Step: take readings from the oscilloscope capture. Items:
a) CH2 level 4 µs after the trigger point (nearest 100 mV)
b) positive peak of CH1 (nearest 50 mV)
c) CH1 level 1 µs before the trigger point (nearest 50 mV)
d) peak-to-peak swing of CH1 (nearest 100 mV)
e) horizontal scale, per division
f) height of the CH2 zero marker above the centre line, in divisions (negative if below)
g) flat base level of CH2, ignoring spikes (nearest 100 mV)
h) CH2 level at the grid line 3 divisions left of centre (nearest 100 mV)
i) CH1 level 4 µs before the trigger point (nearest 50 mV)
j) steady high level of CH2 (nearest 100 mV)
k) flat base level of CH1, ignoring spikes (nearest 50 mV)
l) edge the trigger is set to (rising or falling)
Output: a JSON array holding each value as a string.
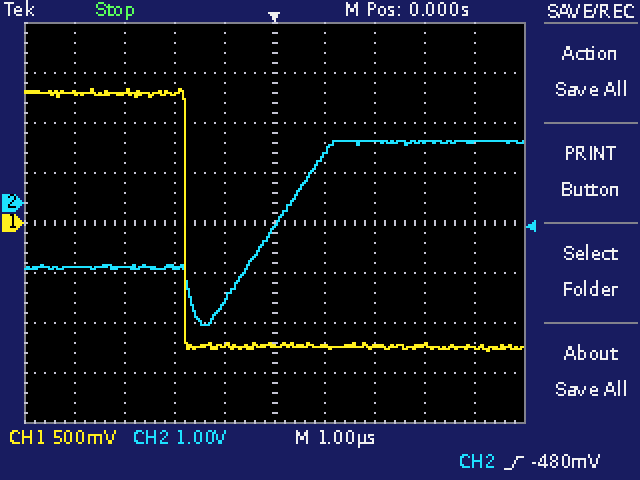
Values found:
["1.2 V", "1.35 V", "-1.20 V", "2.60 V", "1 µs", "+0.4 div", "-1.3 V", "-1.3 V", "1.30 V", "1.2 V", "-1.25 V", "rising"]
